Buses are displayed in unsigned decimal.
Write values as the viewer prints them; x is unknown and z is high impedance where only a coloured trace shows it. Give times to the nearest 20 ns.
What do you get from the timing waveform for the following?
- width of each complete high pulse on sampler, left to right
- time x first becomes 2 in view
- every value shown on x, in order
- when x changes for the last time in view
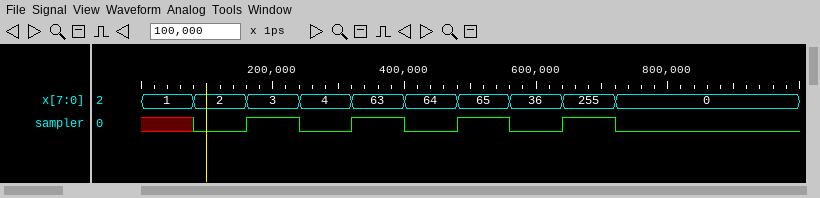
80 ns, 80 ns, 80 ns, 80 ns
80 ns
1, 2, 3, 4, 63, 64, 65, 36, 255, 0
720 ns
